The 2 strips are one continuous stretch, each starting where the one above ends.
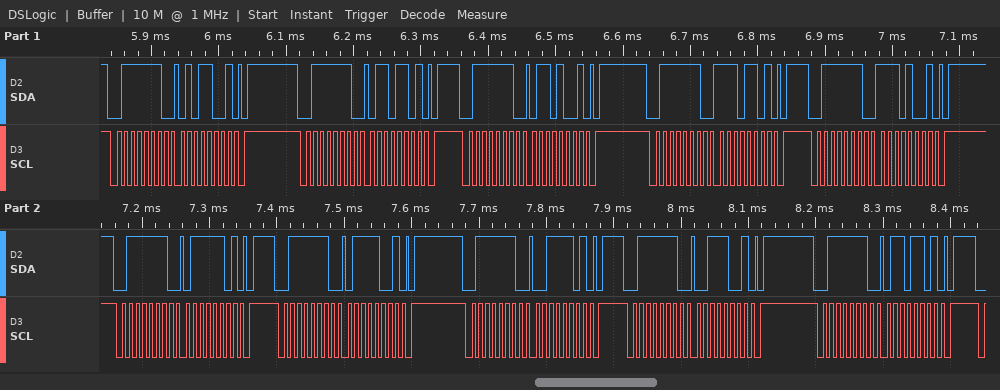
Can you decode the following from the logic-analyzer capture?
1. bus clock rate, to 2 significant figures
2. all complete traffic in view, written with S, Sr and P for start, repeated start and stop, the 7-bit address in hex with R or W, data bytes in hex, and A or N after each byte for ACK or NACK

100 kHz
S 3FW A 59 A P S 3FW A 6D A P S 3FW A 69 A P S 3FW A ED A P S 3FW A E9 A P S 3FW A 7D A P S 3FW A 79 A P S 3FW A 3D A P S 3FW A 39 A P S 3FW A 6D A P
